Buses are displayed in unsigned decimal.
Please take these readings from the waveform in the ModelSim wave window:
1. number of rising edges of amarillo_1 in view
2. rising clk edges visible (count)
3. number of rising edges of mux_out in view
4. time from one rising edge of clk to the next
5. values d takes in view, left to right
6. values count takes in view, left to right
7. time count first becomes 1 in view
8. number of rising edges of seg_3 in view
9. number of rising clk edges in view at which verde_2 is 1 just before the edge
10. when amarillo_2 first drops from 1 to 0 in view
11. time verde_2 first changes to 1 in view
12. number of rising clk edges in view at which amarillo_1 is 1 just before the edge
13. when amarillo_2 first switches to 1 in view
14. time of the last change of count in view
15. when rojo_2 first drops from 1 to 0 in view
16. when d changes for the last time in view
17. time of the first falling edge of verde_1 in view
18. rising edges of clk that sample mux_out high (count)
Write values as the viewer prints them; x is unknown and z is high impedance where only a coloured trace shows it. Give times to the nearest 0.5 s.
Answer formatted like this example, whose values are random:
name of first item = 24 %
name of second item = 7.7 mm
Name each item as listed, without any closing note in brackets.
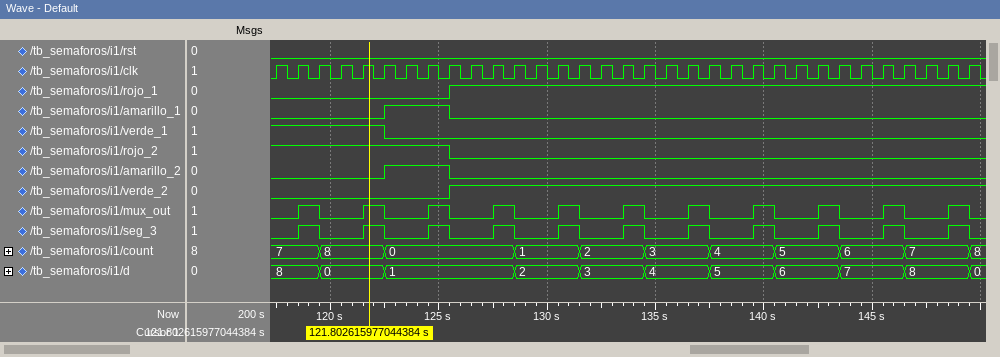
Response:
number of rising edges of amarillo_1 in view = 1
rising clk edges visible = 33
number of rising edges of mux_out in view = 11
time from one rising edge of clk to the next = 1 s
values d takes in view, left to right = 8, 0, 1, 2, 3, 4, 5, 6, 7, 8, 0
values count takes in view, left to right = 7, 8, 0, 1, 2, 3, 4, 5, 6, 7, 8
time count first becomes 1 in view = 128.5 s
number of rising edges of seg_3 in view = 11
number of rising clk edges in view at which verde_2 is 1 just before the edge = 24
when amarillo_2 first drops from 1 to 0 in view = 125.5 s
time verde_2 first changes to 1 in view = 125.5 s
number of rising clk edges in view at which amarillo_1 is 1 just before the edge = 3
when amarillo_2 first switches to 1 in view = 122.5 s
time of the last change of count in view = 149.5 s
when rojo_2 first drops from 1 to 0 in view = 125.5 s
when d changes for the last time in view = 149.5 s
time of the first falling edge of verde_1 in view = 122.5 s
rising edges of clk that sample mux_out high = 11
